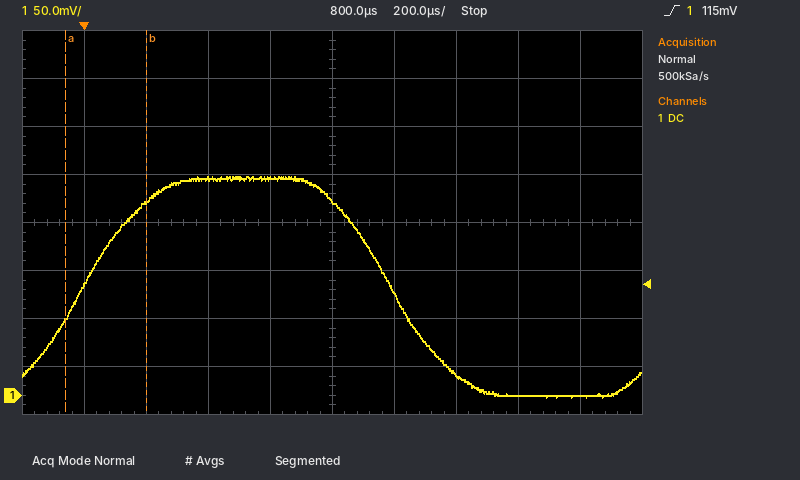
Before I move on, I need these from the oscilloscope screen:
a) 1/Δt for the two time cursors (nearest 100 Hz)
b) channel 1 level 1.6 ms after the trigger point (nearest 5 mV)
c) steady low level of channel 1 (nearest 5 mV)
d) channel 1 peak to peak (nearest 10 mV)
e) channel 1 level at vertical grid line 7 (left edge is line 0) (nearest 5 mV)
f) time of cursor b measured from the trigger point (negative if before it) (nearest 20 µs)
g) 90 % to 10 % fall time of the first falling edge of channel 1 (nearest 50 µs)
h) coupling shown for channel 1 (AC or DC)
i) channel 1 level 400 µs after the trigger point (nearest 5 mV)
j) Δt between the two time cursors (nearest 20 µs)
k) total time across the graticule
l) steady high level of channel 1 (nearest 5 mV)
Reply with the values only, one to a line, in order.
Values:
3.8 kHz
0 mV
0 mV
230 mV
20 mV
+200 µs
400 µs
DC
225 mV
260 µs
2 ms
225 mV
